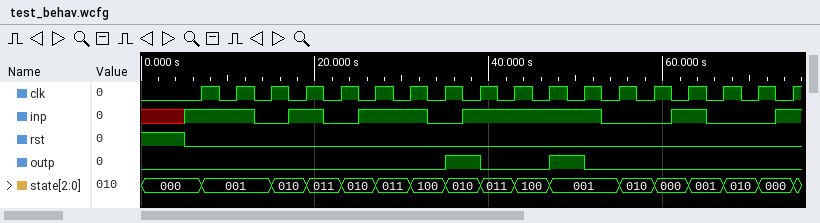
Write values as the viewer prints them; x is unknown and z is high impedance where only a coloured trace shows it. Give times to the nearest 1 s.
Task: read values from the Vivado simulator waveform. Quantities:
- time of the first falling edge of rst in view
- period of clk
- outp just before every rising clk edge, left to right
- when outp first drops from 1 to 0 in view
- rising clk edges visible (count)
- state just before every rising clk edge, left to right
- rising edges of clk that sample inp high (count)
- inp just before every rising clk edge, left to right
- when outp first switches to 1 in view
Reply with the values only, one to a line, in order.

5 s
4 s
0 0 0 0 0 0 0 0 1 0 0 1 0 0 0 0 0 0
39 s
18
000, 001, 001, 010, 011, 010, 011, 100, 010, 011, 100, 001, 001, 010, 000, 001, 010, 000
11
1 1 0 1 0 1 1 0 1 1 1 1 0 0 1 0 0 1
35 s
